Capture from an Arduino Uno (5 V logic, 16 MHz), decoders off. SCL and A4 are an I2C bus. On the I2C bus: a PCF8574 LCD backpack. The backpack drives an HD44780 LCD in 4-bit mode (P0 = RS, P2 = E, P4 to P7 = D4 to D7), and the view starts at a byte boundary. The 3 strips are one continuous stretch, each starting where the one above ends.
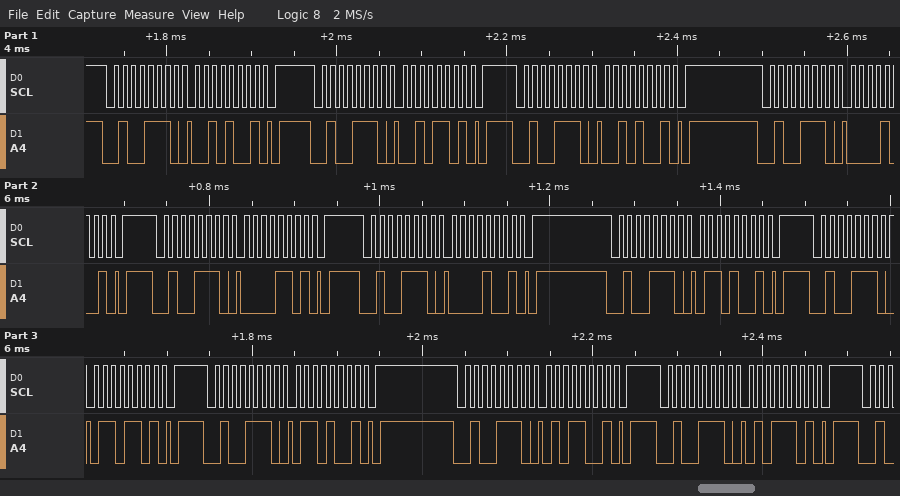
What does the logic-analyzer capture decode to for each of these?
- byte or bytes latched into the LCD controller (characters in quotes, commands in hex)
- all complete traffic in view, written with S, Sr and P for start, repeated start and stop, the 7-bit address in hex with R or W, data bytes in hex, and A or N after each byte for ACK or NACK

' '
S 27W A 29 A P S 27W A 2D A P S 27W A 29 A P S 27W A 09 A P S 27W A 0D A P S 27W A 09 A P S 27W A 69 A P S 27W A 6D A P S 27W A 69 A P S 27W A 59 A P S 27W A 5D A P
